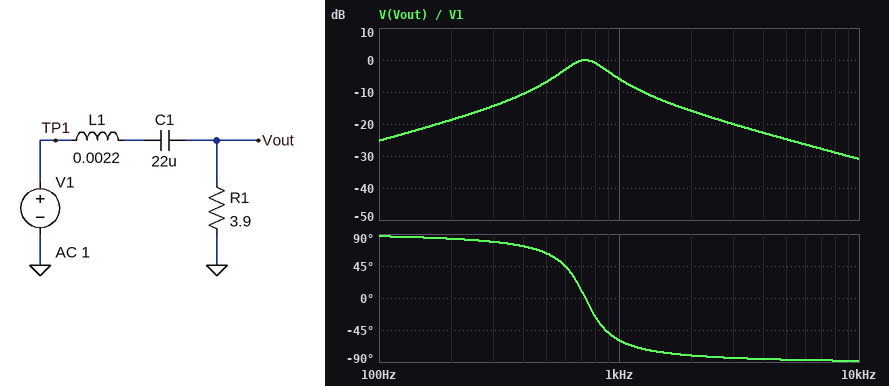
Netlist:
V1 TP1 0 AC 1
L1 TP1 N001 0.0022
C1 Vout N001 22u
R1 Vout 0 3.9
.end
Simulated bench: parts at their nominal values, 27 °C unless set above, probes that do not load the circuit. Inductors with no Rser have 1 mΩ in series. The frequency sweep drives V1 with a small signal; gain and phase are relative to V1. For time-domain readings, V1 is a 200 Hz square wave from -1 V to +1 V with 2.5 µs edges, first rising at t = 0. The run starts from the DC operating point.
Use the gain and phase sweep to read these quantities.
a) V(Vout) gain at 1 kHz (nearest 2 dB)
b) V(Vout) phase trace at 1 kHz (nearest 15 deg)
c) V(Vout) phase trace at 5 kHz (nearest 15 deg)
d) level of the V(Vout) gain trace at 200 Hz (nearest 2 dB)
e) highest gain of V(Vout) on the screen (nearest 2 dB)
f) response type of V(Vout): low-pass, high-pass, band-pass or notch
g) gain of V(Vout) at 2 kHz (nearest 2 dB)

-6 dB
-60 deg
-90 deg
-18 dB
0 dB
band-pass
-16 dB
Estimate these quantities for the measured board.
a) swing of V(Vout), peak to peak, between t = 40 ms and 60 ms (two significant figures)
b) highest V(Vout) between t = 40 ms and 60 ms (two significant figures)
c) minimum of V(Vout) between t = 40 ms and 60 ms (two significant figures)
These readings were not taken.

1.2 V
590 mV
-590 mV
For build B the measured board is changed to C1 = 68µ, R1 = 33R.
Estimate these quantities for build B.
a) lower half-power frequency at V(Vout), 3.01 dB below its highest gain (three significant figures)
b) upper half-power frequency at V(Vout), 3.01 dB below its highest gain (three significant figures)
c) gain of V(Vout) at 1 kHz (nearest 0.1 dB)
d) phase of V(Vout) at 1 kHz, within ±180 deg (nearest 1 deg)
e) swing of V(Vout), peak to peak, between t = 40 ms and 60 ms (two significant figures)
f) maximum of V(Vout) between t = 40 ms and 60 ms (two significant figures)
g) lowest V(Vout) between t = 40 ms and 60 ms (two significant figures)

68.9 Hz
2.46 kHz
-0.5 dB
-19 deg
2.8 V
1.4 V
-1.4 V
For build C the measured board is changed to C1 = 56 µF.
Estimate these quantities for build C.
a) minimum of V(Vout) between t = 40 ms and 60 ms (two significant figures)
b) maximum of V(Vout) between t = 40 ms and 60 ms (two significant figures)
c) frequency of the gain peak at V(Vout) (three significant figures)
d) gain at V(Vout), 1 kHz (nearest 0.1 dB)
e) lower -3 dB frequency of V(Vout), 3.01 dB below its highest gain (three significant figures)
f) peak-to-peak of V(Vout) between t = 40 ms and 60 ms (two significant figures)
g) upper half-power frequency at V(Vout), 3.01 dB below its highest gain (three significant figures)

-740 mV
740 mV
453 Hz
-9.5 dB
334 Hz
1.5 V
616 Hz
